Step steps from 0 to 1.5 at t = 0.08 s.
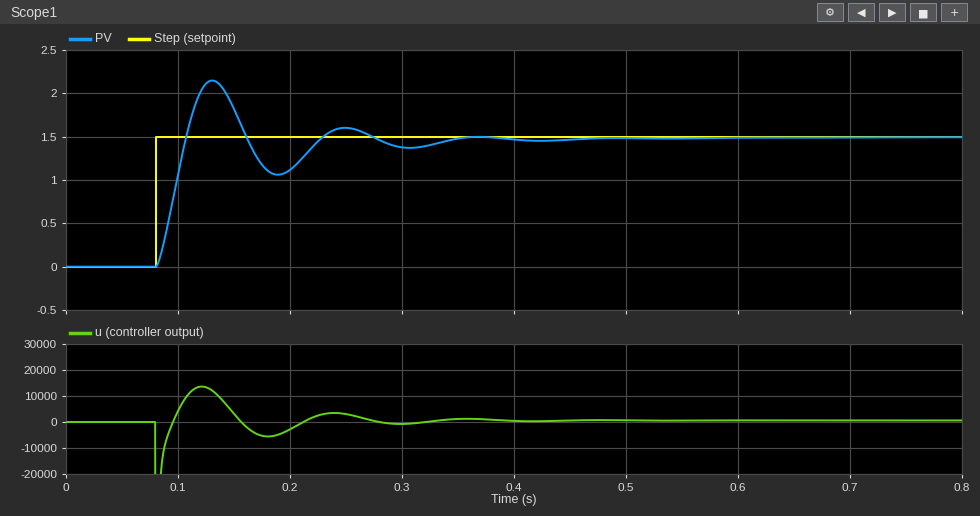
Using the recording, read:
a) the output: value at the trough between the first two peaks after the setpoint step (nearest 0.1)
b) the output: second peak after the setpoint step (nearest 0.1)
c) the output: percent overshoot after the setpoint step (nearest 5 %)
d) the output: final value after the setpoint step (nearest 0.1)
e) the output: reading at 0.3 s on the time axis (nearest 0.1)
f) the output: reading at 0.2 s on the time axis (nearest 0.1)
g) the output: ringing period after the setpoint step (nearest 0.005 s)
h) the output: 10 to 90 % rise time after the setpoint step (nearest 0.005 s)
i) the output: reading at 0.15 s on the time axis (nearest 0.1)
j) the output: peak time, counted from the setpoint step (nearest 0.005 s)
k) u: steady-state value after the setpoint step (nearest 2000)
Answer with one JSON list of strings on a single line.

["1.1", "1.6", "45 %", "1.5", "1.4", "1.1", "0.120 s", "0.020 s", "1.8", "0.050 s", "0"]
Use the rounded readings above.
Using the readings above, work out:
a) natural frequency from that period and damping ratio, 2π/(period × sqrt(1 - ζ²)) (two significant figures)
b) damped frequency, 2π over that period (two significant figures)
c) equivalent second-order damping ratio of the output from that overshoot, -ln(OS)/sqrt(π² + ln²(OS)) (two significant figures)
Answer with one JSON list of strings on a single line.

["54 rad/s", "52 rad/s", "0.25"]
